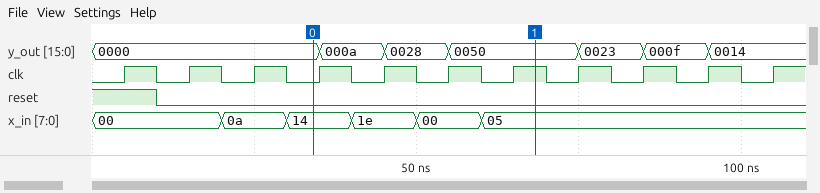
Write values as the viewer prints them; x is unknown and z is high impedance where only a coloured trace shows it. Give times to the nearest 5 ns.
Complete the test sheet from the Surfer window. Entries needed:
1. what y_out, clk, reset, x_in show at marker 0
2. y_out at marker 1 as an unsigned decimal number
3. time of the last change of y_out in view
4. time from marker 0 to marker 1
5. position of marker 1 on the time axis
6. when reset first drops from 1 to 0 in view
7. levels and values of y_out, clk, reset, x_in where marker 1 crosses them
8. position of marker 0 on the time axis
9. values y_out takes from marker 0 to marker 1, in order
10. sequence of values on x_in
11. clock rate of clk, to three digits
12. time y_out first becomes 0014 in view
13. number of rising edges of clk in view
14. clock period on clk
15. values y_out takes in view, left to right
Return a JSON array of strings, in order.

["y_out=0000, clk=0, reset=0, x_in=14", "80", "95 ns", "35 ns", "70 ns", "10 ns", "y_out=0050, clk=1, reset=0, x_in=05", "35 ns", "0000, 000a, 0028, 0050", "00, 0a, 14, 1e, 00, 05", "100 MHz", "95 ns", "11", "10 ns", "0000, 000a, 0028, 0050, 0023, 000f, 0014"]
